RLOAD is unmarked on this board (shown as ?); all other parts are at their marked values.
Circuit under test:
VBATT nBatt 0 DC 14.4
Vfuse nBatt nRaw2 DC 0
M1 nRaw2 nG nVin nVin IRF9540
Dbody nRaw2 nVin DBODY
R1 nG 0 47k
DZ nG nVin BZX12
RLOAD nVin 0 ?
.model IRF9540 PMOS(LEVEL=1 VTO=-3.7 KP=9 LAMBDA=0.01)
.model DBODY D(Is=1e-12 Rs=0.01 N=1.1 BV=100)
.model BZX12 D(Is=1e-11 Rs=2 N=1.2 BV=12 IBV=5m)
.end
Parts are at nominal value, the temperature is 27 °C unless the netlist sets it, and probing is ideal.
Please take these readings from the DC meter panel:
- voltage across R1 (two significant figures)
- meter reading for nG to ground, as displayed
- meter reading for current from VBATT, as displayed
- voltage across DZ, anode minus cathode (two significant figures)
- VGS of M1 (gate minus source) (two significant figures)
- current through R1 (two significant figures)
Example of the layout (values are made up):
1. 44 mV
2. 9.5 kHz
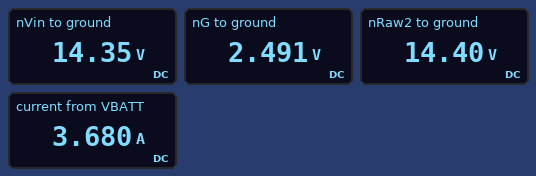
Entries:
1. 2.5 V
2. 2.491 V
3. 3.680 A
4. -12 V
5. -12 V
6. 53 µA
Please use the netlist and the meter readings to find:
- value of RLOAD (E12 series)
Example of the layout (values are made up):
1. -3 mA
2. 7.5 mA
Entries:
1. 3.9 Ω
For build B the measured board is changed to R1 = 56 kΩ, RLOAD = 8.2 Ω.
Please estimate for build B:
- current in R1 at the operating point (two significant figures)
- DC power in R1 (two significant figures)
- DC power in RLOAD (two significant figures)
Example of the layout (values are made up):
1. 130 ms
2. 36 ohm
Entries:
1. 45 µA
2. 110 µW
3. 25 W
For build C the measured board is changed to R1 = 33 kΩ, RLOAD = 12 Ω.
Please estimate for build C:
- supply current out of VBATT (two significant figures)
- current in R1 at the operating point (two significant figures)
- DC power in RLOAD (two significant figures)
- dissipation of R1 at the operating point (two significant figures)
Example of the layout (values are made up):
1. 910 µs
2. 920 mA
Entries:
1. 1.2 A
2. 76 µA
3. 17 W
4. 190 µW
